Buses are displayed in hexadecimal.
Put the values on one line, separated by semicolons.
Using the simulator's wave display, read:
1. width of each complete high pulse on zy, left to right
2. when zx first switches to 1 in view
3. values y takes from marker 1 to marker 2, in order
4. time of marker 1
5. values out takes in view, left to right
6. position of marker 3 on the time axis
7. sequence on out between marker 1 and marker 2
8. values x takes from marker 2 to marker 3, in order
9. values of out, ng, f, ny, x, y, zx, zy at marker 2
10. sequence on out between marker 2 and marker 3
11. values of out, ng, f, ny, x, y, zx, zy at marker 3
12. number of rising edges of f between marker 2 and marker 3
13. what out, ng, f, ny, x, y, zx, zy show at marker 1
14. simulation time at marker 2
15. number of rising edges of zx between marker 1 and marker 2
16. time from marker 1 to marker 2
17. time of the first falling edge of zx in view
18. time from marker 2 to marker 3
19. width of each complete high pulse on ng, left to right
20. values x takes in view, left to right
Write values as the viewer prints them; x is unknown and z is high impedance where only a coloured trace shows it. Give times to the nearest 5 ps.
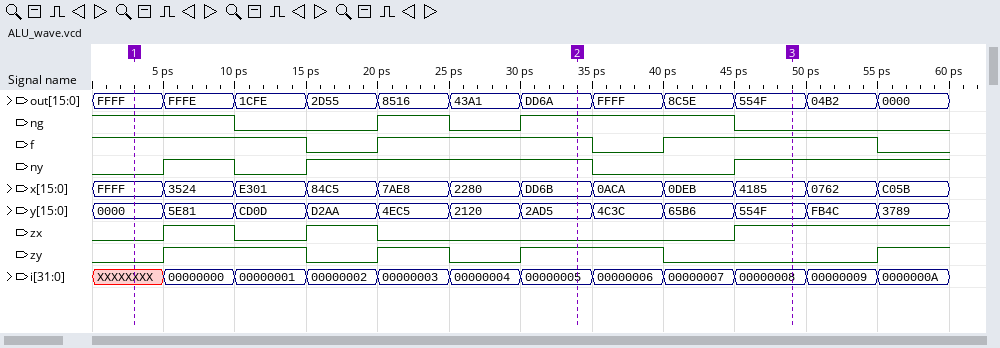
10 ps, 5 ps, 10 ps; 5 ps; 0000, 5E81, CD0D, D2AA, 4EC5, 2120, 2AD5; 5 ps; FFFF, FFFE, 1CFE, 2D55, 8516, 43A1, DD6A, FFFF, 8C5E, 554F, 04B2, 0000; 50 ps; FFFF, FFFE, 1CFE, 2D55, 8516, 43A1, DD6A; DD6B, 0ACA, 0DEB, 4185; out=DD6A, ng=1, f=1, ny=1, x=DD6B, y=2AD5, zx=0, zy=1; DD6A, FFFF, 8C5E, 554F; out=554F, ng=0, f=1, ny=1, x=4185, y=554F, zx=1, zy=0; 1; out=FFFF, ng=1, f=1, ny=0, x=FFFF, y=0000, zx=0, zy=0; 35 ps; 2; 30 ps; 10 ps; 15 ps; 5 ps, 15 ps; FFFF, 3524, E301, 84C5, 7AE8, 2280, DD6B, 0ACA, 0DEB, 4185, 0762, C05B
